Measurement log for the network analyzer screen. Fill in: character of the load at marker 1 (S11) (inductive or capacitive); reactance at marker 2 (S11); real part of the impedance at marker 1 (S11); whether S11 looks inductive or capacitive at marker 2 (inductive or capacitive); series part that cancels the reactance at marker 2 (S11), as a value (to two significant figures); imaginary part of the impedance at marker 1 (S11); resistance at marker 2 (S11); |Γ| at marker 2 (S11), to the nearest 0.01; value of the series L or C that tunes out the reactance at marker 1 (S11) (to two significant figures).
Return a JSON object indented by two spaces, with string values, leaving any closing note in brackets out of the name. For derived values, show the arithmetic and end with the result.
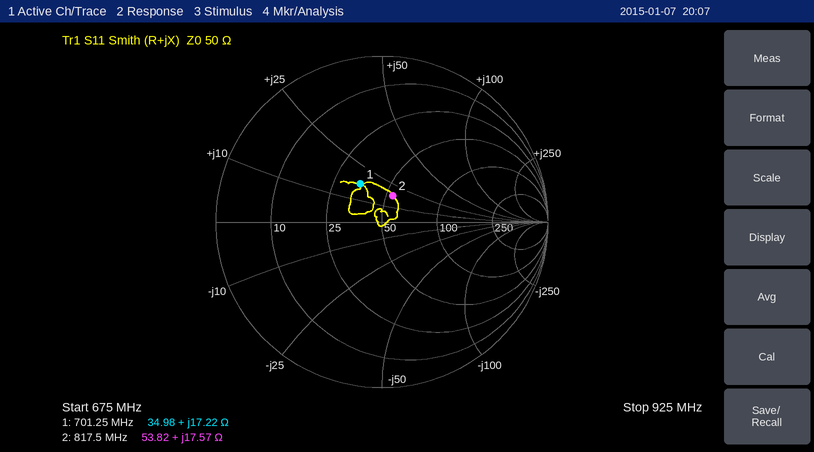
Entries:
{
  "character of the load at marker 1 (S11)": "inductive",
  "reactance at marker 2": "+17.57 Ω",
  "real part of the impedance at marker 1": "34.98 Ω",
  "whether S11 looks inductive or capacitive at marker 2": "inductive",
  "series part that cancels the reactance at marker 2 (S11), as a value": "C = 1/(2π × 817.5 MHz × 17.57 Ω) ≈ 11 pF",
  "imaginary part of the impedance at marker 1": "+17.22 Ω",
  "resistance at marker 2": "53.82 Ω",
  "|Γ| at marker 2 (S11), to the nearest 0.01": "0.17",
  "value of the series L or C that tunes out the reactance at marker 1 (S11)": "C = 1/(2π × 701.25 MHz × 17.22 Ω) ≈ 13 pF"
}
